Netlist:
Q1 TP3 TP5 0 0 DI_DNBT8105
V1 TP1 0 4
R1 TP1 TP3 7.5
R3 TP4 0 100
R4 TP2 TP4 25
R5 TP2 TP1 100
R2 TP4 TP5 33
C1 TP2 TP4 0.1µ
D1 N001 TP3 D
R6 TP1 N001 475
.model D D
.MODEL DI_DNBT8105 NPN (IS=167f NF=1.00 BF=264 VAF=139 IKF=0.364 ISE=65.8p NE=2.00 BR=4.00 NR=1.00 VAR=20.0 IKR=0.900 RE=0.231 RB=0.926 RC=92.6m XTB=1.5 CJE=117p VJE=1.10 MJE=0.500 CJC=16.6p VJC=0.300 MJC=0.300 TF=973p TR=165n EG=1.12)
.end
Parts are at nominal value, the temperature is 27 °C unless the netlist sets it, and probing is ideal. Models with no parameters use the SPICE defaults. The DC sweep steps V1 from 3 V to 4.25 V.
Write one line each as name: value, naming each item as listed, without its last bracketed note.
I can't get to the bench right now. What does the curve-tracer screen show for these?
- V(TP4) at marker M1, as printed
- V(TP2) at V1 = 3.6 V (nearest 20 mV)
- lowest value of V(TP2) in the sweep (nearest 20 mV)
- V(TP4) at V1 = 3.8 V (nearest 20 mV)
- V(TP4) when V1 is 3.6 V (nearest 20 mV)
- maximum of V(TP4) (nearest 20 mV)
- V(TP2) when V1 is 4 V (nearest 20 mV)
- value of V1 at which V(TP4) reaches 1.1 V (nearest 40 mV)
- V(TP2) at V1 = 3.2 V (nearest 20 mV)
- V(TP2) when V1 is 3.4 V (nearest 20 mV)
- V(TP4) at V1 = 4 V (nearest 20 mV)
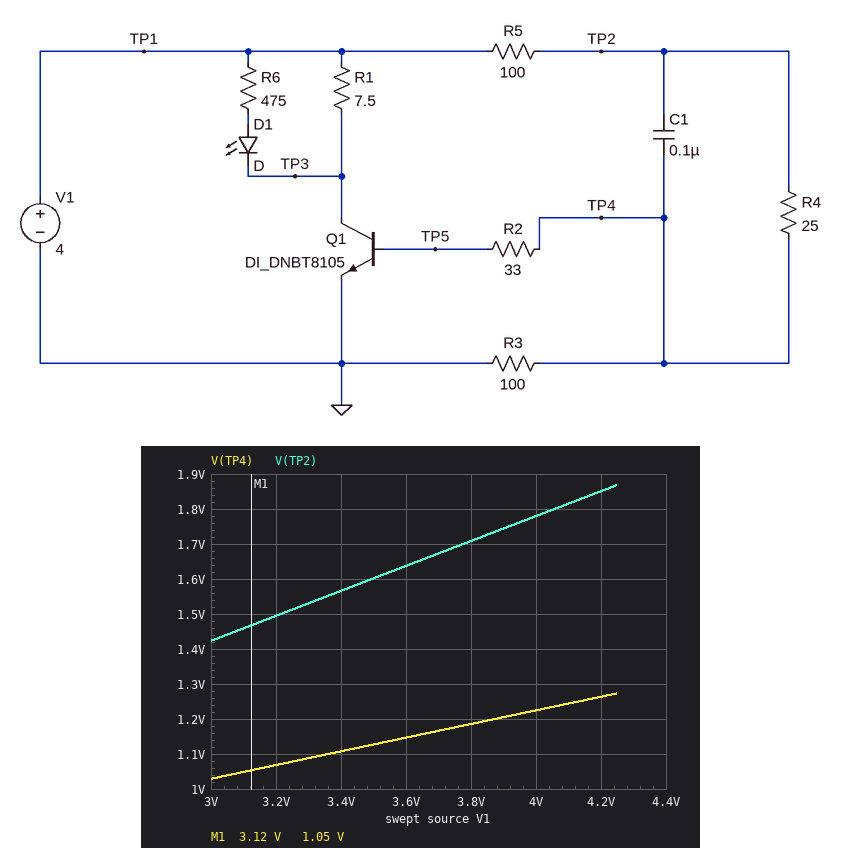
V(TP4) at marker M1, as printed: 1.05 V
V(TP2) at V1 = 3.6 V: 1.64 V
lowest value of V(TP2) in the sweep: 1.42 V
V(TP4) at V1 = 3.8 V: 1.18 V
V(TP4) when V1 is 3.6 V: 1.14 V
maximum of V(TP4): 1.28 V
V(TP2) when V1 is 4 V: 1.78 V
value of V1 at which V(TP4) reaches 1.1 V: 3.36 V
V(TP2) at V1 = 3.2 V: 1.50 V
V(TP2) when V1 is 3.4 V: 1.56 V
V(TP4) at V1 = 4 V: 1.22 V
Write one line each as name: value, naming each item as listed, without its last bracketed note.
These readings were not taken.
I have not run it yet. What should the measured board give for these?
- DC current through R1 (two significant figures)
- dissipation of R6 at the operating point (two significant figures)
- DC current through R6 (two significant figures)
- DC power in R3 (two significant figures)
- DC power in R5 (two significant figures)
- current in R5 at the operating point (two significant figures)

DC current through R1: 500 mA
dissipation of R6 at the operating point: 19 mW
DC current through R6: 6.4 mA
DC power in R3: 15 mW
DC power in R5: 49 mW
current in R5 at the operating point: 22 mA
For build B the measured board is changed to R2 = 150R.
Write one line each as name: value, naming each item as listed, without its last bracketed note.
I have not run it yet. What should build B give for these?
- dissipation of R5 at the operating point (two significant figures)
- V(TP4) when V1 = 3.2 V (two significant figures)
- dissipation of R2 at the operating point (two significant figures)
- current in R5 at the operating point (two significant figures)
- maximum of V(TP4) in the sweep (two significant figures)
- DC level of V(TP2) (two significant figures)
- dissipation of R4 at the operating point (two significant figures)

dissipation of R5 at the operating point: 39 mW
V(TP4) when V1 = 3.2 V: 1.3 V
dissipation of R2 at the operating point: 2.9 mW
current in R5 at the operating point: 20 mA
maximum of V(TP4) in the sweep: 1.6 V
DC level of V(TP2): 2.0 V
dissipation of R4 at the operating point: 9.7 mW
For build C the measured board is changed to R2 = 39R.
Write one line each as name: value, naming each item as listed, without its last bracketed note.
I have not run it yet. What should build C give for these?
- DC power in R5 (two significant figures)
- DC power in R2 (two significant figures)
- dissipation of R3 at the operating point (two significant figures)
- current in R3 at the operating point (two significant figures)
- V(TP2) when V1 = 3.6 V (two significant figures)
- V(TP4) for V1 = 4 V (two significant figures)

DC power in R5: 48 mW
DC power in R2: 3.4 mW
dissipation of R3 at the operating point: 16 mW
current in R3 at the operating point: 13 mA
V(TP2) when V1 = 3.6 V: 1.7 V
V(TP4) for V1 = 4 V: 1.3 V
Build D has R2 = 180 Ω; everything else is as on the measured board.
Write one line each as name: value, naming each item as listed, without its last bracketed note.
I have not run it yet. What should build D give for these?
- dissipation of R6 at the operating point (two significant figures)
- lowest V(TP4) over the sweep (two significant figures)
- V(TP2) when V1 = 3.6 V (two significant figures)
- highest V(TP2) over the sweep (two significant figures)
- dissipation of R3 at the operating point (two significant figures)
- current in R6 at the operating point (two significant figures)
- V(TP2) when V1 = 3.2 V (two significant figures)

dissipation of R6 at the operating point: 13 mW
lowest V(TP4) over the sweep: 1.2 V
V(TP2) when V1 = 3.6 V: 1.9 V
highest V(TP2) over the sweep: 2.2 V
dissipation of R3 at the operating point: 24 mW
current in R6 at the operating point: 5.2 mA
V(TP2) when V1 = 3.2 V: 1.7 V
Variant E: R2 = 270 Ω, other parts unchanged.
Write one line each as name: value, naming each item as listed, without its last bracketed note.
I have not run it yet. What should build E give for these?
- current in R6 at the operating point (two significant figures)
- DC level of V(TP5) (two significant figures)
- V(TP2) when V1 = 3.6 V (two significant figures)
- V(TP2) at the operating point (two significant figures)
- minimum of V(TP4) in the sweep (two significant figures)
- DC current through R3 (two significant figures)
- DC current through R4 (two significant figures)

current in R6 at the operating point: 4.0 mA
DC level of V(TP5): 840 mV
V(TP2) when V1 = 3.6 V: 1.9 V
V(TP2) at the operating point: 2.1 V
minimum of V(TP4) in the sweep: 1.2 V
DC current through R3: 16 mA
DC current through R4: 19 mA
